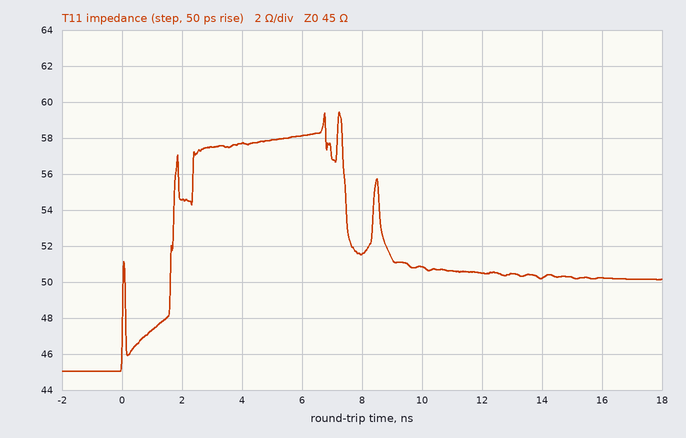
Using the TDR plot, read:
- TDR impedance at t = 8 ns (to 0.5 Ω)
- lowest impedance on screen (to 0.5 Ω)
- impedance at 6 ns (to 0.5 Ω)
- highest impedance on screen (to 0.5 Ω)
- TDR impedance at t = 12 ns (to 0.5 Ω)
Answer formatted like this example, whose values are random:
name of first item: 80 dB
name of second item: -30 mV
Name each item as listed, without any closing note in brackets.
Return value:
TDR impedance at t = 8 ns: 51.5 Ω
lowest impedance on screen: 45.0 Ω
impedance at 6 ns: 58.0 Ω
highest impedance on screen: 59.5 Ω
TDR impedance at t = 12 ns: 50.5 Ω
